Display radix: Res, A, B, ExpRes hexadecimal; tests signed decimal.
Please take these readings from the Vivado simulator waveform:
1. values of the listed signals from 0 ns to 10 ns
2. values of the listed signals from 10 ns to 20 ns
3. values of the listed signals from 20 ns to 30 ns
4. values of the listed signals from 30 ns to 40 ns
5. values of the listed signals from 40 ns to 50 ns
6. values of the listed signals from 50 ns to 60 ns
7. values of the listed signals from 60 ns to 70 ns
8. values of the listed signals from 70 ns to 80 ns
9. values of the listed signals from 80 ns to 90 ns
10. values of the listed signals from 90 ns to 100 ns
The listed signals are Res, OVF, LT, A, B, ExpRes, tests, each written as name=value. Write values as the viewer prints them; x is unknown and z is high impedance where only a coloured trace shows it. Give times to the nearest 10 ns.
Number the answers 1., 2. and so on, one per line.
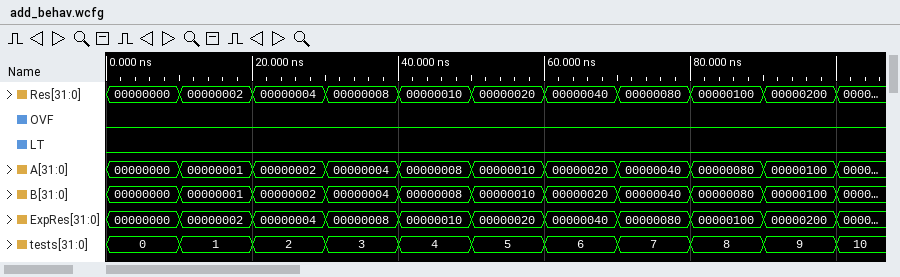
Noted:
1. Res=00000000, OVF=0, LT=0, A=00000000, B=00000000, ExpRes=00000000, tests=0
2. Res=00000002, OVF=0, LT=0, A=00000001, B=00000001, ExpRes=00000002, tests=1
3. Res=00000004, OVF=0, LT=0, A=00000002, B=00000002, ExpRes=00000004, tests=2
4. Res=00000008, OVF=0, LT=0, A=00000004, B=00000004, ExpRes=00000008, tests=3
5. Res=00000010, OVF=0, LT=0, A=00000008, B=00000008, ExpRes=00000010, tests=4
6. Res=00000020, OVF=0, LT=0, A=00000010, B=00000010, ExpRes=00000020, tests=5
7. Res=00000040, OVF=0, LT=0, A=00000020, B=00000020, ExpRes=00000040, tests=6
8. Res=00000080, OVF=0, LT=0, A=00000040, B=00000040, ExpRes=00000080, tests=7
9. Res=00000100, OVF=0, LT=0, A=00000080, B=00000080, ExpRes=00000100, tests=8
10. Res=00000200, OVF=0, LT=0, A=00000100, B=00000100, ExpRes=00000200, tests=9
